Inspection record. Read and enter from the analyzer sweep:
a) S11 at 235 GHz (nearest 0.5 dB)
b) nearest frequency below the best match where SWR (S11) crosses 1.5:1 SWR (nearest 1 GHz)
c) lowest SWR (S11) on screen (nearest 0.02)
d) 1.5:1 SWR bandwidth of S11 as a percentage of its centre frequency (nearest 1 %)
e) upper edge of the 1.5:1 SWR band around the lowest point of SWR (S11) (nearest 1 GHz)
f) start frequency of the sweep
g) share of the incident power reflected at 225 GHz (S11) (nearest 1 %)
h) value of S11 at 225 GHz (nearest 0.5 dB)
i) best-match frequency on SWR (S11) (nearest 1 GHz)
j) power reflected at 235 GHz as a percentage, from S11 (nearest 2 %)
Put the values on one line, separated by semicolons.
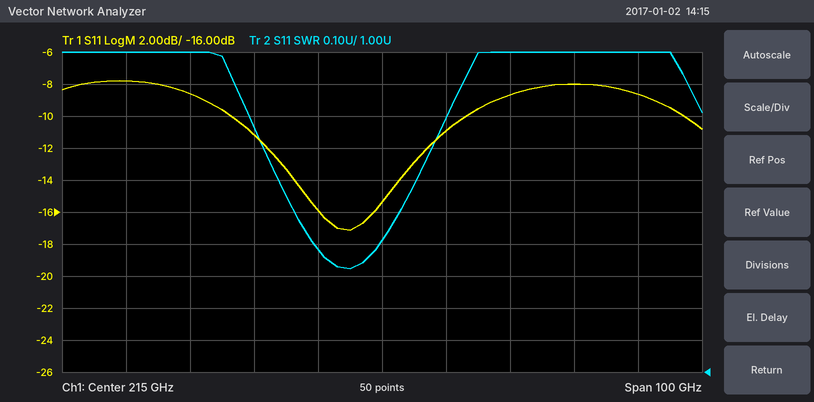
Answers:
-8.5 dB; 201 GHz; 1.32; 8 %; 218 GHz; 165 GHz; 8 %; -11.0 dB; 210 GHz; 14 %
